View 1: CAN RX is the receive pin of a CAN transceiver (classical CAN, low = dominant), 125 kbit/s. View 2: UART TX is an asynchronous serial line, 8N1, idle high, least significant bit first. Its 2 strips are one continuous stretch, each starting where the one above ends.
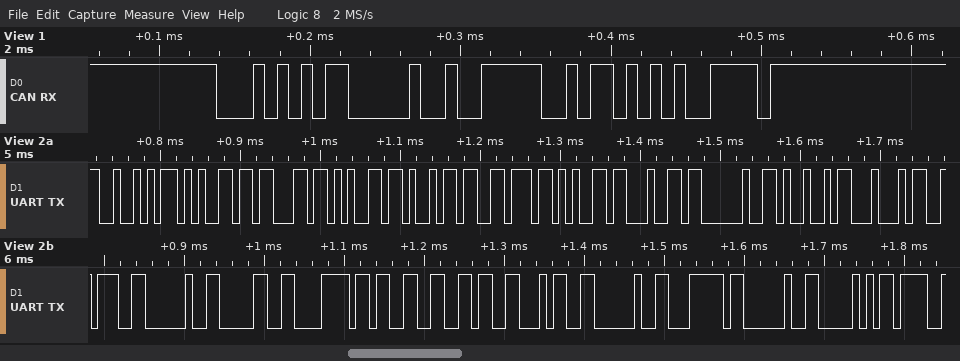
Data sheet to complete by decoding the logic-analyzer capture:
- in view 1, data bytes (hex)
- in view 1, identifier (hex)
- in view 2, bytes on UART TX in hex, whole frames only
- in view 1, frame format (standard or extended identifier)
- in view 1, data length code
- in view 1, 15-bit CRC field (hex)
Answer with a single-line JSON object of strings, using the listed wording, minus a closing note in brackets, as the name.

{"in view 1, data bytes": "3E", "in view 1, identifier": "0x156", "in view 2, bytes on UART TX in hex, whole frames only": "52 65 63 65 69 76 65 64 20 49 44 3A 20 30 78 33 36 34 20 7C 20 50", "in view 1, frame format": "standard", "in view 1, data length code": "1", "in view 1, 15-bit CRC field": "0x5AA7"}
